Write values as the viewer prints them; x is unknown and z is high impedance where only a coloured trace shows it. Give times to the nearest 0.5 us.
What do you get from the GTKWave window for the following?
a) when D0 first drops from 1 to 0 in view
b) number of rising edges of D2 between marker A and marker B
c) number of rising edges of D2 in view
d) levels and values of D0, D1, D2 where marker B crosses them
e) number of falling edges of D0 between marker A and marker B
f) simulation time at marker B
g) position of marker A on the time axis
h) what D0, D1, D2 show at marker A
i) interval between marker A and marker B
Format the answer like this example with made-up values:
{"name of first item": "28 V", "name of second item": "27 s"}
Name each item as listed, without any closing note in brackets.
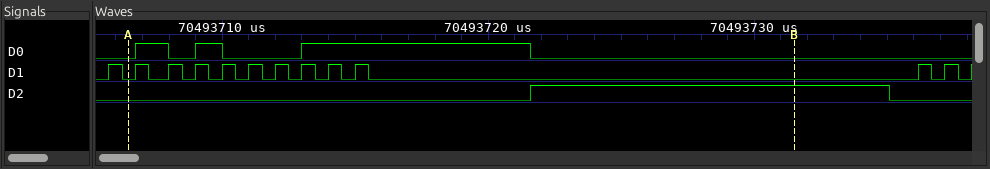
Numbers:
{"when D0 first drops from 1 to 0 in view": "70493708 us", "number of rising edges of D2 between marker A and marker B": "1", "number of rising edges of D2 in view": "1", "levels and values of D0, D1, D2 where marker B crosses them": "D0=0, D1=0, D2=1", "number of falling edges of D0 between marker A and marker B": "3", "simulation time at marker B": "70493731.5 us", "position of marker A on the time axis": "70493706.5 us", "what D0, D1, D2 show at marker A": "D0=0, D1=0, D2=0", "interval between marker A and marker B": "25 us"}
